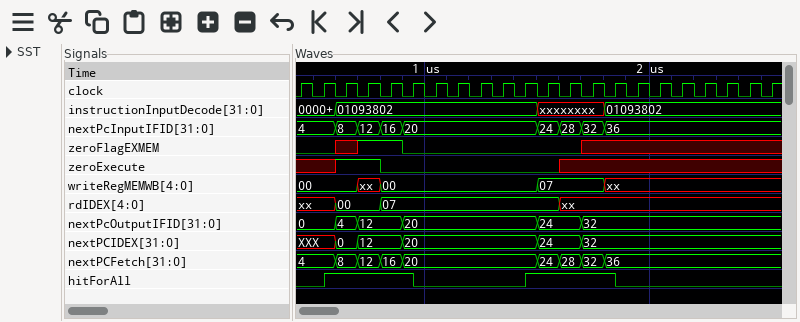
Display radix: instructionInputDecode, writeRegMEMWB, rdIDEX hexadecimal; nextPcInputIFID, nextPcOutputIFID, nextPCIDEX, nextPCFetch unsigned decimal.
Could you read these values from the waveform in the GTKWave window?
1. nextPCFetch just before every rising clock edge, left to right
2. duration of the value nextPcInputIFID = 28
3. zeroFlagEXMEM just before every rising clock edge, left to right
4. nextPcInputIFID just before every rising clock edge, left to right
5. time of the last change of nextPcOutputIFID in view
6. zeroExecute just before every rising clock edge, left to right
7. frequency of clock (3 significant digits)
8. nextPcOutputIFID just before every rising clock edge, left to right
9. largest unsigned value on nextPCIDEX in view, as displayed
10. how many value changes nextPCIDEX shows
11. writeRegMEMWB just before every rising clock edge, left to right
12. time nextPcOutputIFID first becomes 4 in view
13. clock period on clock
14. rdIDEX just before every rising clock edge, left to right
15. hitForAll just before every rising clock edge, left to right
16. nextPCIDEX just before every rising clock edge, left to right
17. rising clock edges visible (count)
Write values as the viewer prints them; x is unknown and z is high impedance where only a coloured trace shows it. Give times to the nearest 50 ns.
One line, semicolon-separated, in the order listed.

4, 4, 8, 12, 16, 20, 20, 20, 20, 20, 20, 24, 28, 32, 36, 36, 36, 36, 36, 36, 36, 36; 100 ns; 0 0 x 1 1 0 0 0 0 0 0 0 0 x x x x x x x x x; 4, 4, 8, 12, 16, 20, 20, 20, 20, 20, 20, 24, 28, 32, 36, 36, 36, 36, 36, 36, 36, 36; 1700 ns; x x 1 1 0 0 0 0 0 0 0 0 x x x x x x x x x x; 10.0 MHz; 0, 0, 4, 12, 12, 20, 20, 20, 20, 20, 20, 24, 24, 32, 32, 32, 32, 32, 32, 32, 32, 32; 32; 5; 00, 00, 00, xx, 00, 00, 00, 00, 00, 00, 00, 07, 07, 07, xx, xx, xx, xx, xx, xx, xx, xx; 600 ns; 100 ns; xx, xx, 00, 00, 07, 07, 07, 07, 07, 07, 07, 07, xx, xx, xx, xx, xx, xx, xx, xx, xx, xx; 0 0 1 1 1 1 0 0 0 0 0 1 1 1 1 0 0 0 0 0 0 0; XXX, XXX, 0, 12, 12, 20, 20, 20, 20, 20, 20, 24, 24, 32, 32, 32, 32, 32, 32, 32, 32, 32; 22
